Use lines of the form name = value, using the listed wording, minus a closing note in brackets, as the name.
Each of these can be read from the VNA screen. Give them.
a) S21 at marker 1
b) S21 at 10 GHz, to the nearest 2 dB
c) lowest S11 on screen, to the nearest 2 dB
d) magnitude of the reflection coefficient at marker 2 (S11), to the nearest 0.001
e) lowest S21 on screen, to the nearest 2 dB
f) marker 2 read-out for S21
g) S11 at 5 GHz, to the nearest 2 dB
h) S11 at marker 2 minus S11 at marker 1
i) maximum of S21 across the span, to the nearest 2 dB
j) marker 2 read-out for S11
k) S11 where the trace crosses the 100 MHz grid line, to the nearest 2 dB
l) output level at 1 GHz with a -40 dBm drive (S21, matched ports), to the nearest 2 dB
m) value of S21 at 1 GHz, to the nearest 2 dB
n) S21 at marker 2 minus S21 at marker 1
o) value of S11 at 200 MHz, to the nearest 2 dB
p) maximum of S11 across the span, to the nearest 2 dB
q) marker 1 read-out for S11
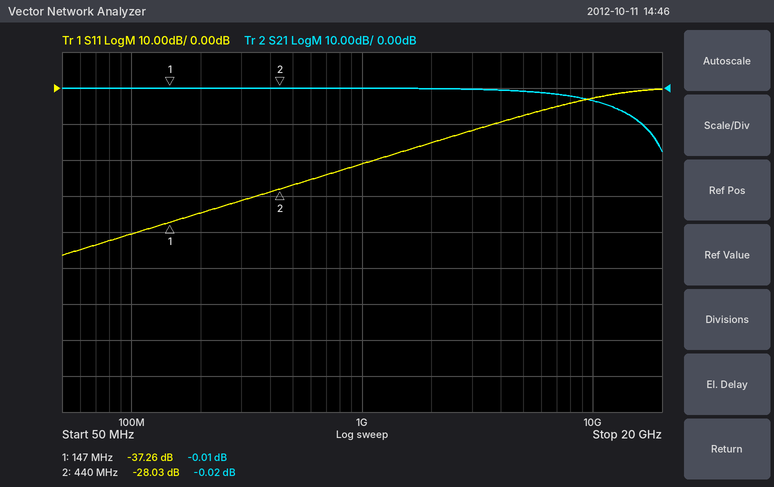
S21 at marker 1 = -0.01 dB
S21 at 10 GHz, to the nearest 2 dB = -4 dB
lowest S11 on screen, to the nearest 2 dB = -46 dB
magnitude of the reflection coefficient at marker 2 (S11), to the nearest 0.001 = 0.040
lowest S21 on screen, to the nearest 2 dB = -18 dB
marker 2 read-out for S21 = -0.02 dB
S11 at 5 GHz, to the nearest 2 dB = -8 dB
S11 at marker 2 minus S11 at marker 1 = 9.23 dB
maximum of S21 across the span, to the nearest 2 dB = 0 dB
marker 2 read-out for S11 = -28.03 dB
S11 where the trace crosses the 100 MHz grid line, to the nearest 2 dB = -40 dB
output level at 1 GHz with a -40 dBm drive (S21, matched ports), to the nearest 2 dB = -40 dBm
value of S21 at 1 GHz, to the nearest 2 dB = 0 dB
S21 at marker 2 minus S21 at marker 1 = -0.01 dB
value of S11 at 200 MHz, to the nearest 2 dB = -34 dB
maximum of S11 across the span, to the nearest 2 dB = 0 dB
marker 1 read-out for S11 = -37.26 dB
